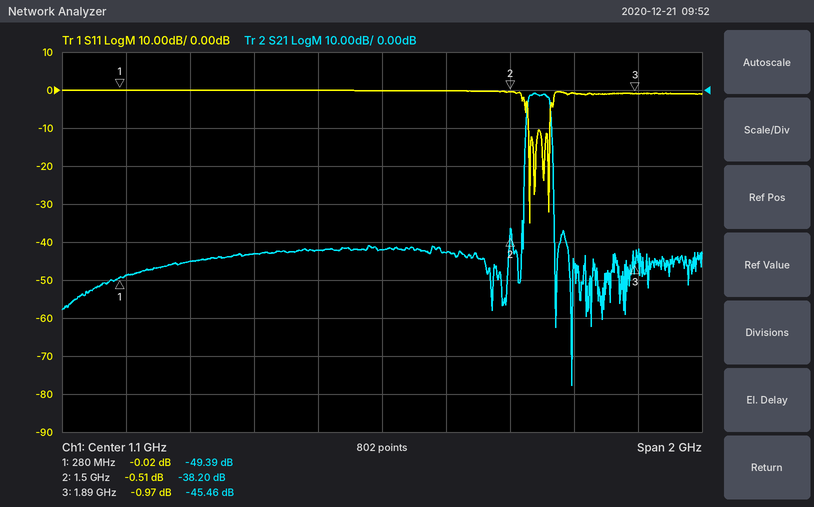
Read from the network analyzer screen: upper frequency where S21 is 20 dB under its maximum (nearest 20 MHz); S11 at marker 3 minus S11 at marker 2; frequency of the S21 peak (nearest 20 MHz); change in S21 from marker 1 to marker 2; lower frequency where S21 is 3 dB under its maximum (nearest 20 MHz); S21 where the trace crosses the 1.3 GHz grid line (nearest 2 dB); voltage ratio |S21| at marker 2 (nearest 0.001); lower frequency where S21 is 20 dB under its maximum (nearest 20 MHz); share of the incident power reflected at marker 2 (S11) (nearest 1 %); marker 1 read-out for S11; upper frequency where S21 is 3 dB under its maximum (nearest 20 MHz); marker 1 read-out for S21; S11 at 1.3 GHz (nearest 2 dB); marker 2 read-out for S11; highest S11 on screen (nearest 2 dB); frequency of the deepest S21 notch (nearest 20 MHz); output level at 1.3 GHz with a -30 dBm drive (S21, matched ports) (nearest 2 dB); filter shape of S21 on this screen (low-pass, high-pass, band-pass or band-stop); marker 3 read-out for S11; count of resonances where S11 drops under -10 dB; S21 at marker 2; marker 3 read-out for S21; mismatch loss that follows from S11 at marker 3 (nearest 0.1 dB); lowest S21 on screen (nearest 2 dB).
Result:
1.64 GHz
-0.46 dB
1.58 GHz
11.19 dB
1.56 GHz
-42 dB
0.012
1.54 GHz
89 %
-0.02 dB
1.62 GHz
-49.39 dB
0 dB
-0.51 dB
0 dB
1.70 GHz
-72 dBm
band-pass
-0.97 dB
4
-38.20 dB
-45.46 dB
7.0 dB
-78 dB
